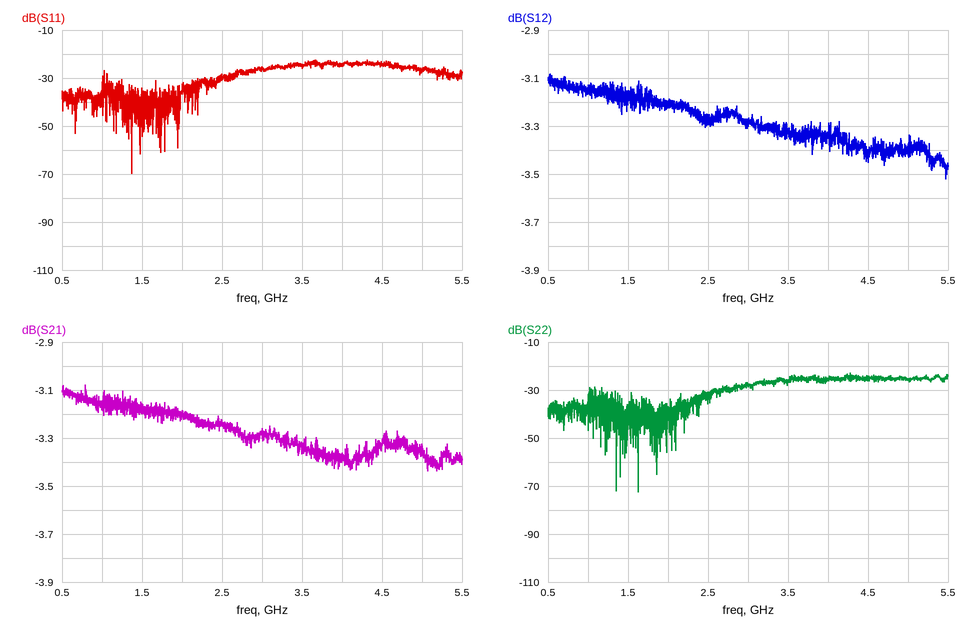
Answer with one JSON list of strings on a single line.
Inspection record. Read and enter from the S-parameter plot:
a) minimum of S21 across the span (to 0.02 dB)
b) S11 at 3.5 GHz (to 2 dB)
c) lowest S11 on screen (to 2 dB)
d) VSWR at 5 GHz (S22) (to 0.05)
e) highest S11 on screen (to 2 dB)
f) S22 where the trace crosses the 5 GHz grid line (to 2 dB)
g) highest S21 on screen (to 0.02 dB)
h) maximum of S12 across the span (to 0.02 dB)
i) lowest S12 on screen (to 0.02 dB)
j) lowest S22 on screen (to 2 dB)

["-3.44 dB", "-24 dB", "-70 dB", "1.10", "-22 dB", "-26 dB", "-3.08 dB", "-3.08 dB", "-3.52 dB", "-72 dB"]
